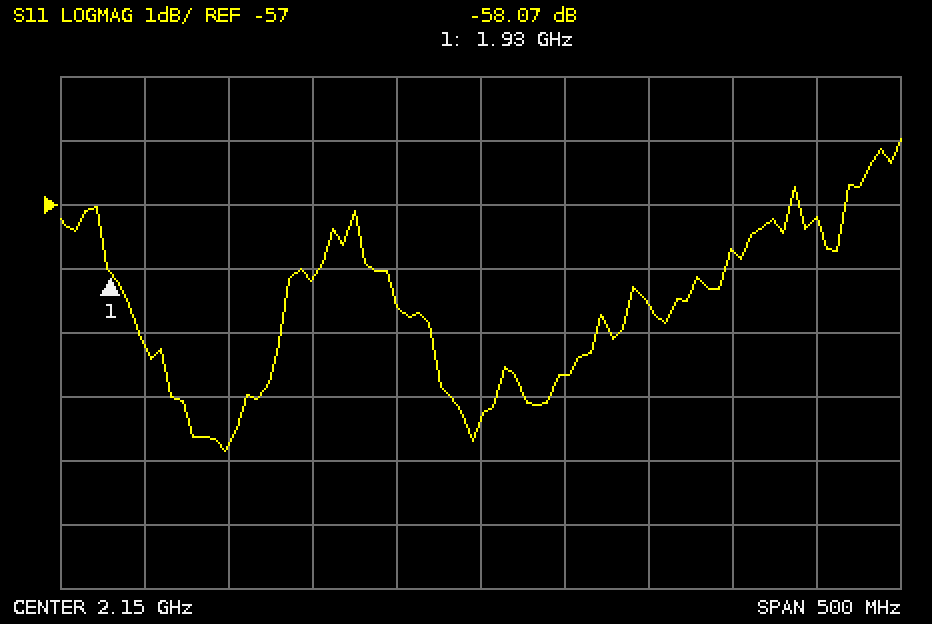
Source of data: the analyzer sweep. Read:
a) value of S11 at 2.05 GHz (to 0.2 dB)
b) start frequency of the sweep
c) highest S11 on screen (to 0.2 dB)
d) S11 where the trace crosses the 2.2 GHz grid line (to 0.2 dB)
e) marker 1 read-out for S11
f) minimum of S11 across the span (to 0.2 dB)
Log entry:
-58.2 dB
1.9 GHz
-56.0 dB
-59.6 dB
-58.07 dB
-60.8 dB
